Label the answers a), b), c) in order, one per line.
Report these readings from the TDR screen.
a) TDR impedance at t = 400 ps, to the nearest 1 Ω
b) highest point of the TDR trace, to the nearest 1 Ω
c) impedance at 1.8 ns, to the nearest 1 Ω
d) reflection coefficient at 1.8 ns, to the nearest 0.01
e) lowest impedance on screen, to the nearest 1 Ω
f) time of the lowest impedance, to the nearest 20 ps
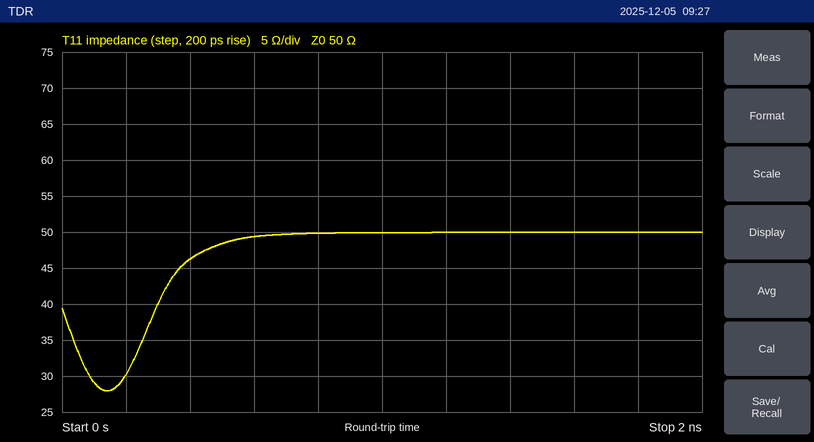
a) 46 Ω
b) 50 Ω
c) 50 Ω
d) 0.00
e) 28 Ω
f) 140 ps
